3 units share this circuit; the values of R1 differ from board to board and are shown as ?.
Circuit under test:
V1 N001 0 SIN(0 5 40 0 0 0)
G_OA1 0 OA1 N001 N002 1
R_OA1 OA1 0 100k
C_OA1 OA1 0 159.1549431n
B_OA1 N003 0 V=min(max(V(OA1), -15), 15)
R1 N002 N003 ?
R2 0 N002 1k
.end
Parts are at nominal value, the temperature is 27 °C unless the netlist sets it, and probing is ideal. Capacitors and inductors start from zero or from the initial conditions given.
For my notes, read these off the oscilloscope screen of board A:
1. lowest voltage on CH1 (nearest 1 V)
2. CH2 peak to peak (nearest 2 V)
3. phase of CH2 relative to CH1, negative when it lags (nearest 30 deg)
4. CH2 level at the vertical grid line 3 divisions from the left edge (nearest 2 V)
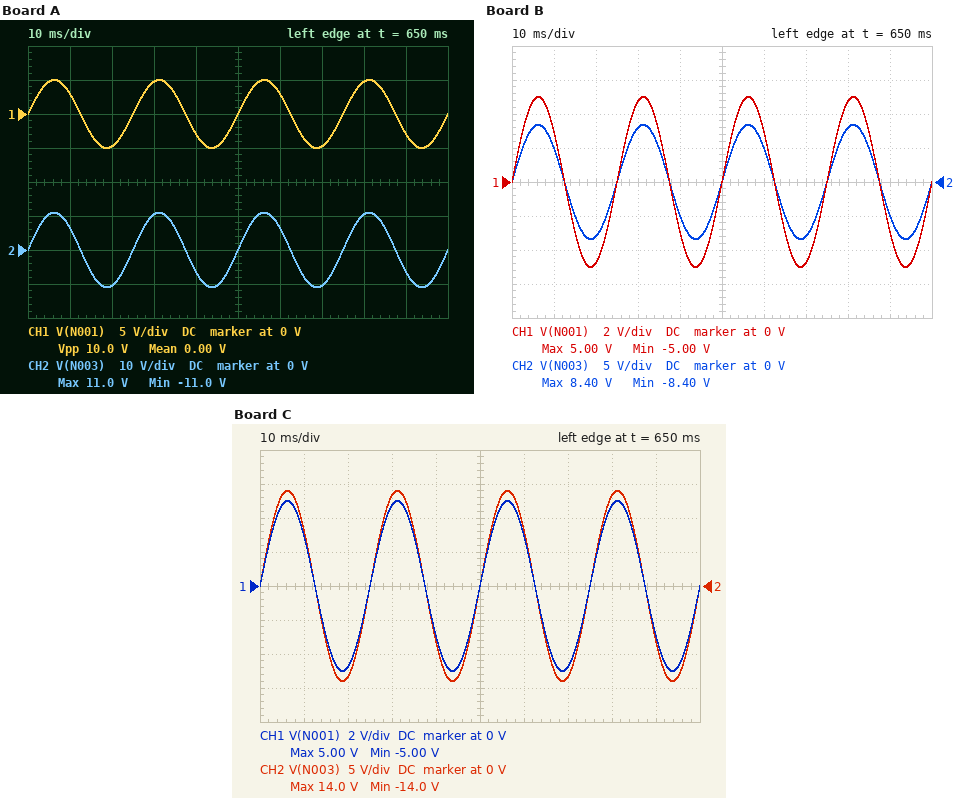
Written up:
-5 V
22 V
0 deg
10 V
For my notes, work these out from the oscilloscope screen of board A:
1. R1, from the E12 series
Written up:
1.2 kΩ
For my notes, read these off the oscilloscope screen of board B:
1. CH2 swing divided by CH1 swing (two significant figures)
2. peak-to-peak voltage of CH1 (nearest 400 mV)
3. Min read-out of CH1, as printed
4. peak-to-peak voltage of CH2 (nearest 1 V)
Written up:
1.7
10.0 V
-5.00 V
17 V
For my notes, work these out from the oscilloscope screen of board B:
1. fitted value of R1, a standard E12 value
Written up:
680 Ω
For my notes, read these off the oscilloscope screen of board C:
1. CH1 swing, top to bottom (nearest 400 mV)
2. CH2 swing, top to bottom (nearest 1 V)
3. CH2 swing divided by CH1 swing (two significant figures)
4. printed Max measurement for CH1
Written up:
10.0 V
28 V
2.8
5.00 V
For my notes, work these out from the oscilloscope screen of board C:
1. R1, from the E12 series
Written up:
1.8 kΩ
